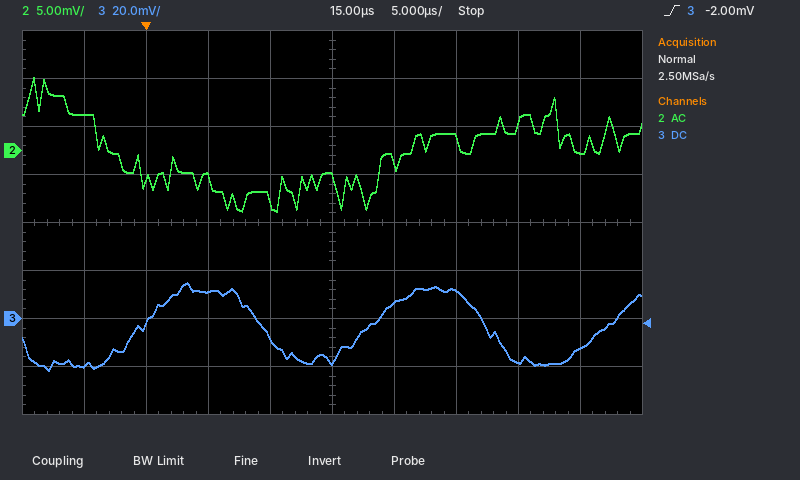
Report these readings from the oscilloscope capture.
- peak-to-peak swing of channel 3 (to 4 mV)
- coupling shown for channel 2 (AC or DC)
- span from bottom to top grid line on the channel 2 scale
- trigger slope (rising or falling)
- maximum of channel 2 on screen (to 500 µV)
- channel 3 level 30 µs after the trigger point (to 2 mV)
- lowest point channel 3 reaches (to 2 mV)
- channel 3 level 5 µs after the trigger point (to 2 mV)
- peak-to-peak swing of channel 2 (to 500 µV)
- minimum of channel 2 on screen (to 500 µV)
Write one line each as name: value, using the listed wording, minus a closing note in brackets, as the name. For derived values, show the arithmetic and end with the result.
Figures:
peak-to-peak swing of channel 3: 36 mV
coupling shown for channel 2: AC
span from bottom to top grid line on the channel 2 scale: 40 mV
trigger slope: rising
maximum of channel 2 on screen: 7.5 mV
channel 3 level 30 µs after the trigger point: -18 mV
lowest point channel 3 reaches: -22 mV
channel 3 level 5 µs after the trigger point: 12 mV
peak-to-peak swing of channel 2: 7.5 mV − (-6.5 mV) = 14.0 mV
minimum of channel 2 on screen: -6.5 mV
